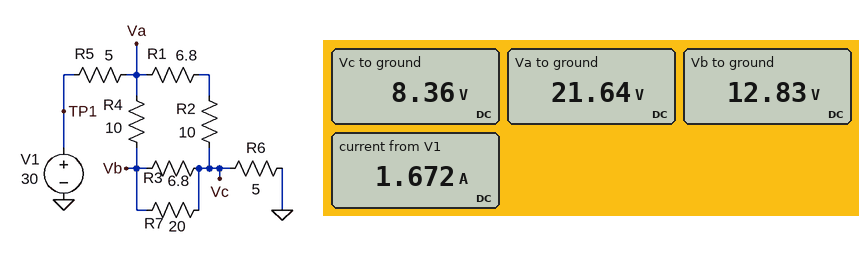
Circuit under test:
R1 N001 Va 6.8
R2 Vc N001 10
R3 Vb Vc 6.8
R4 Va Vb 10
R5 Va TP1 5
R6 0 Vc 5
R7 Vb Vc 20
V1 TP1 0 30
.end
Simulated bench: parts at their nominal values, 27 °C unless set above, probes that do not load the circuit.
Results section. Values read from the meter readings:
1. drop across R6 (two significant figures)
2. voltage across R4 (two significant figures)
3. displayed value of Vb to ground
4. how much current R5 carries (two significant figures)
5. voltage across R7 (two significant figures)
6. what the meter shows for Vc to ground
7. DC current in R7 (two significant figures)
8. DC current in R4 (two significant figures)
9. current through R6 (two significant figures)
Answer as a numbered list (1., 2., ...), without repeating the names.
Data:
1. 8.4 V
2. 8.8 V
3. 12.83 V
4. 1.7 A
5. 4.5 V
6. 8.36 V
7. 220 mA
8. 880 mA
9. 1.7 A
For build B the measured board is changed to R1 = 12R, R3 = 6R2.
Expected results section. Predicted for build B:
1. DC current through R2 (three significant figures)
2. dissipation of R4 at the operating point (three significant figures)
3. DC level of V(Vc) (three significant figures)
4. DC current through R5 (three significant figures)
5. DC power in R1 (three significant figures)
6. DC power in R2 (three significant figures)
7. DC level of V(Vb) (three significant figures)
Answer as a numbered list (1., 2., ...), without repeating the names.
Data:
1. 639 mA
2. 9.11 W
3. 7.97 V
4. 1.59 A
5. 4.90 W
6. 4.09 W
7. 12.5 V
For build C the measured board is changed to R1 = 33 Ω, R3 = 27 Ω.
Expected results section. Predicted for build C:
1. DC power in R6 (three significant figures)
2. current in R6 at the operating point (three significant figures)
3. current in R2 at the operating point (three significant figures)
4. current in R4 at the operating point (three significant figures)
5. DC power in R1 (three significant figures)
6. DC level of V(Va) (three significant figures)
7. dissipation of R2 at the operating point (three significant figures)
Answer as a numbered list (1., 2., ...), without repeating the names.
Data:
1. 7.60 W
2. 1.23 A
3. 411 mA
4. 822 mA
5. 5.57 W
6. 23.8 V
7. 1.69 W
